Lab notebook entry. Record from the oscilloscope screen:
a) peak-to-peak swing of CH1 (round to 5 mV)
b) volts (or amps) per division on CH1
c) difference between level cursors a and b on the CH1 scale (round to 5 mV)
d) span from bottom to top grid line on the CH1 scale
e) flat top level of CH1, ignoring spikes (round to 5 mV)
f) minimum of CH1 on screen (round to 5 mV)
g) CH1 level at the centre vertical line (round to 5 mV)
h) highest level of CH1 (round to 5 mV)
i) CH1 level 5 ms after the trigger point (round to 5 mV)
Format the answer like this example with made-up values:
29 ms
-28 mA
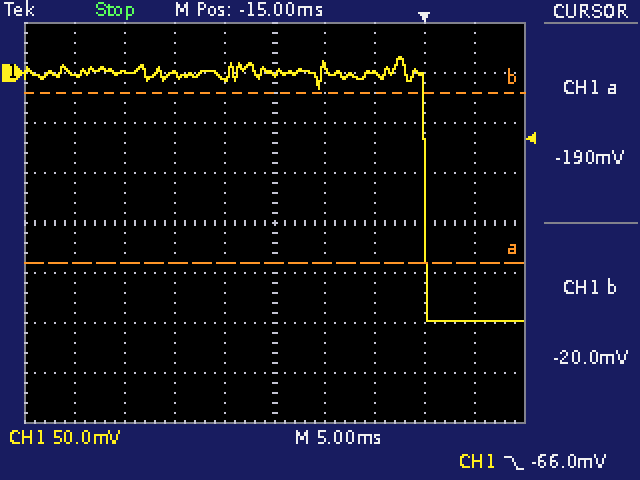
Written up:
265 mV
50 mV
170 mV
400 mV
0 mV
-250 mV
0 mV
15 mV
-250 mV
